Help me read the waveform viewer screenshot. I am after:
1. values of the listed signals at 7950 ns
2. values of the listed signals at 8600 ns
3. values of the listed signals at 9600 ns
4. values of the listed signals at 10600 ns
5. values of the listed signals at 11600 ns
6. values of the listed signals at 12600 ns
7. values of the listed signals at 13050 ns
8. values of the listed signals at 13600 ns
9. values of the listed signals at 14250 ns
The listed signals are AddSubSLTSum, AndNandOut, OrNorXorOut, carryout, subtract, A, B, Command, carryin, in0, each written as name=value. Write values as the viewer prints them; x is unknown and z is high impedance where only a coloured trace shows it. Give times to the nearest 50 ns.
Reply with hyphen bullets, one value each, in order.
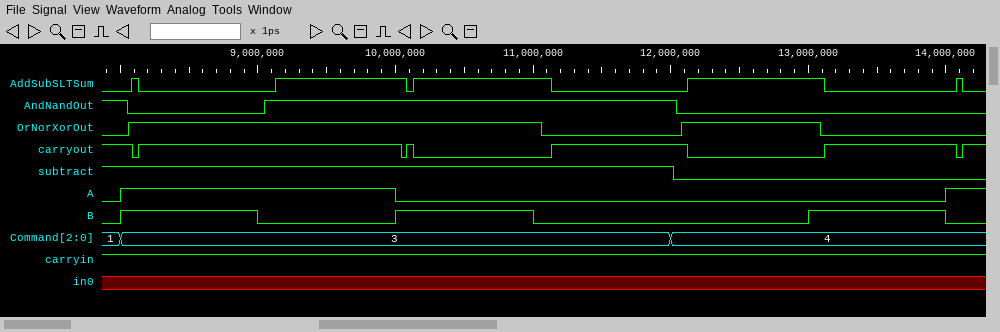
- AddSubSLTSum=0, AndNandOut=1, OrNorXorOut=0, carryout=1, subtract=1, A=0, B=0, Command=1, carryin=1, in0=x
- AddSubSLTSum=0, AndNandOut=0, OrNorXorOut=1, carryout=1, subtract=1, A=1, B=1, Command=3, carryin=1, in0=x
- AddSubSLTSum=1, AndNandOut=1, OrNorXorOut=1, carryout=1, subtract=1, A=1, B=0, Command=3, carryin=1, in0=x
- AddSubSLTSum=1, AndNandOut=1, OrNorXorOut=1, carryout=0, subtract=1, A=0, B=1, Command=3, carryin=1, in0=x
- AddSubSLTSum=0, AndNandOut=1, OrNorXorOut=0, carryout=1, subtract=1, A=0, B=0, Command=3, carryin=1, in0=x
- AddSubSLTSum=1, AndNandOut=0, OrNorXorOut=1, carryout=0, subtract=0, A=0, B=0, Command=4, carryin=1, in0=x
- AddSubSLTSum=1, AndNandOut=0, OrNorXorOut=1, carryout=0, subtract=0, A=0, B=1, Command=4, carryin=1, in0=x
- AddSubSLTSum=0, AndNandOut=0, OrNorXorOut=0, carryout=1, subtract=0, A=0, B=1, Command=4, carryin=1, in0=x
- AddSubSLTSum=0, AndNandOut=0, OrNorXorOut=0, carryout=1, subtract=0, A=1, B=0, Command=4, carryin=1, in0=x
